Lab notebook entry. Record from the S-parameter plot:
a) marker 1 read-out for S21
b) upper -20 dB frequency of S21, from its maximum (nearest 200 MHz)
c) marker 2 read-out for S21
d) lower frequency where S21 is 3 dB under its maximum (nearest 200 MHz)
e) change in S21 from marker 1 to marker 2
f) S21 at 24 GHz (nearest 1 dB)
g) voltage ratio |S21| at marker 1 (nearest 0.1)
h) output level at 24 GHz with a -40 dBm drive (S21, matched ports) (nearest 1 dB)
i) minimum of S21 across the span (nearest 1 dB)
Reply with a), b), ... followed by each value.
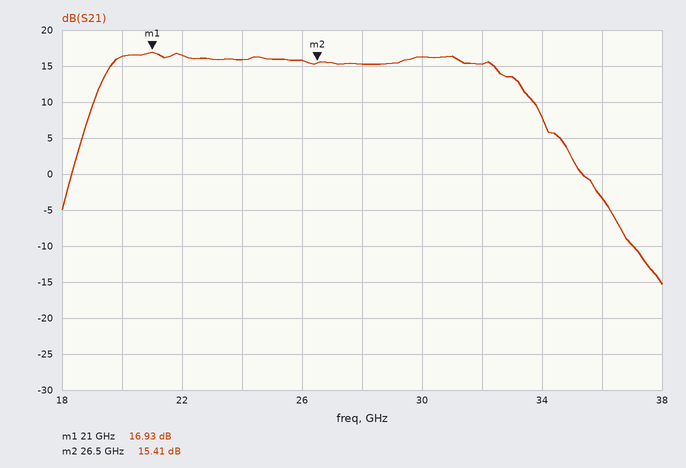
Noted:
a) 16.93 dB
b) 36.0 GHz
c) 15.41 dB
d) 19.4 GHz
e) -1.52 dB
f) 16 dB
g) 7.0
h) -24 dBm
i) -15 dB
